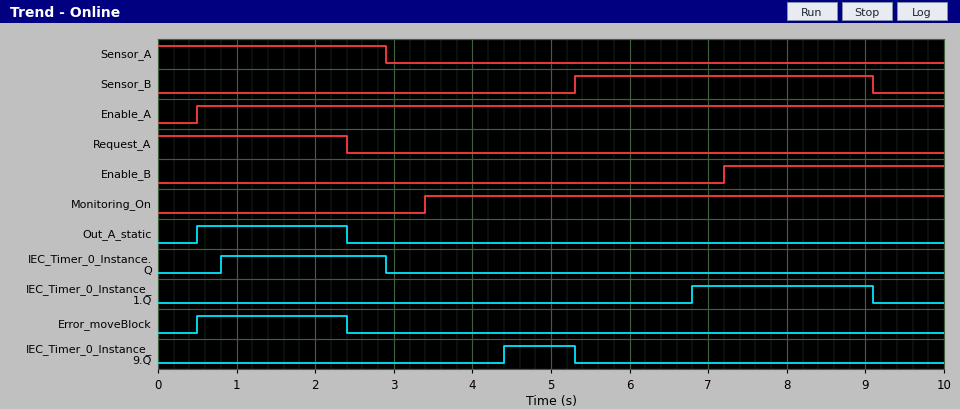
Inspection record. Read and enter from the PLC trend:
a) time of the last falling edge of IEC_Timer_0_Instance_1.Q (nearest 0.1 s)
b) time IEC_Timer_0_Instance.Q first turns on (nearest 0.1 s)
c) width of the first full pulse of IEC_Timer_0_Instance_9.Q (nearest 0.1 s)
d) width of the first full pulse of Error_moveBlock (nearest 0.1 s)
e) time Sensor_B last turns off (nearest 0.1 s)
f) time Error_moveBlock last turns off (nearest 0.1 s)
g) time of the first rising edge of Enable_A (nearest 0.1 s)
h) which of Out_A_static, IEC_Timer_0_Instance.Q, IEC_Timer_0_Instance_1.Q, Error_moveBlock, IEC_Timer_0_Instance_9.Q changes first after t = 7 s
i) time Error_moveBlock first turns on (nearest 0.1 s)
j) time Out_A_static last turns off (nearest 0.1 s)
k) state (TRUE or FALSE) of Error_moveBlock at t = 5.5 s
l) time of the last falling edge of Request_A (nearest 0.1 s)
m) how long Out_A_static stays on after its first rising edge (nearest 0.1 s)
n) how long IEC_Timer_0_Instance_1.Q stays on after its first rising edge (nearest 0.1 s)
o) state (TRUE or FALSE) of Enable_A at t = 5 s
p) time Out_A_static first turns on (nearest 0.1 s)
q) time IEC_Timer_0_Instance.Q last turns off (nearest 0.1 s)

9.1 s
0.8 s
0.9 s
1.9 s
9.1 s
2.4 s
0.5 s
IEC_Timer_0_Instance_1.Q
0.5 s
2.4 s
FALSE
2.4 s
1.9 s
2.3 s
TRUE
0.5 s
2.9 s
